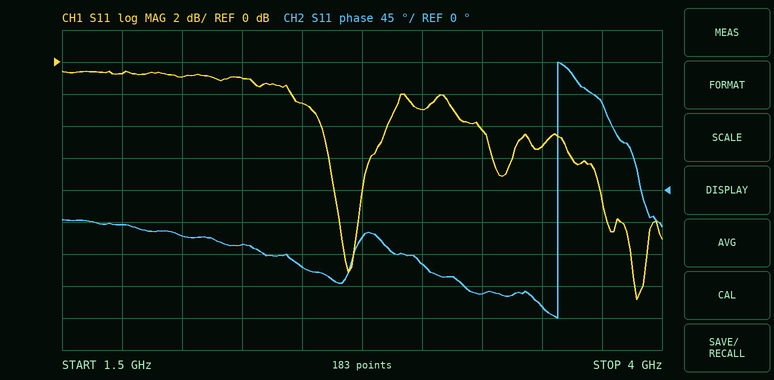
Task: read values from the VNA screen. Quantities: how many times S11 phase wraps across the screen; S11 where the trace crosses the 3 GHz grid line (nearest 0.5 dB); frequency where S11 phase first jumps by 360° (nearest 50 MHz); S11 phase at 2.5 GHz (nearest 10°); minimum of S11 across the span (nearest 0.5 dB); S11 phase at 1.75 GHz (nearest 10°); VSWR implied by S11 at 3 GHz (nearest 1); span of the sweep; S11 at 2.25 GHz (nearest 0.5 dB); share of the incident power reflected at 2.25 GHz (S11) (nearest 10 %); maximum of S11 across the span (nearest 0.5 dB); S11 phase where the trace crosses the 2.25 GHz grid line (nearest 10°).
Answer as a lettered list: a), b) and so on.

a) 1
b) -3.0 dB
c) 3.55 GHz
d) -110°
e) -15.0 dB
f) -50°
g) 6
h) 2.5 GHz
i) -1.0 dB
j) 80 %
k) -0.5 dB
l) -80°
